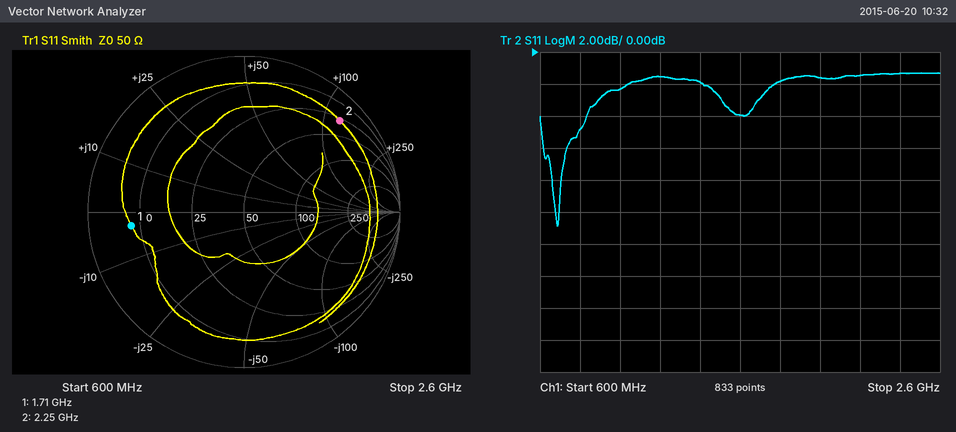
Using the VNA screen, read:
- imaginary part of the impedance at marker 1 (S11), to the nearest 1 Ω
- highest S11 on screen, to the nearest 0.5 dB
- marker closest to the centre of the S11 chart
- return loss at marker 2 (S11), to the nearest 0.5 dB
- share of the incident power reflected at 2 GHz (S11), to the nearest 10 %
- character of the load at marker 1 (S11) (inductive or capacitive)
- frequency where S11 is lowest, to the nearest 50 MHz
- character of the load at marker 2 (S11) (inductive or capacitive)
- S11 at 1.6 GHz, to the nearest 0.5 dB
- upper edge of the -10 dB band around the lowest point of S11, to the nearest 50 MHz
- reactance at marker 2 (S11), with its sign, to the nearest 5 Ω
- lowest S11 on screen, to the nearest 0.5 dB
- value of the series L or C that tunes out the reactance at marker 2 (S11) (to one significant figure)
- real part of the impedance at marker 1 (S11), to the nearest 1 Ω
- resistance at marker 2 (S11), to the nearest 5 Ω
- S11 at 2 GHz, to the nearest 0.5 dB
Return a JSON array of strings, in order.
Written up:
["-3 Ω", "-1.5 dB", "marker 1", "1.5 dB", "70 %", "capacitive", "700 MHz", "inductive", "-4.0 dB", "700 MHz", "+120 Ω", "-11.0 dB", "600 fF", "8 Ω", "30 Ω", "-1.5 dB"]
